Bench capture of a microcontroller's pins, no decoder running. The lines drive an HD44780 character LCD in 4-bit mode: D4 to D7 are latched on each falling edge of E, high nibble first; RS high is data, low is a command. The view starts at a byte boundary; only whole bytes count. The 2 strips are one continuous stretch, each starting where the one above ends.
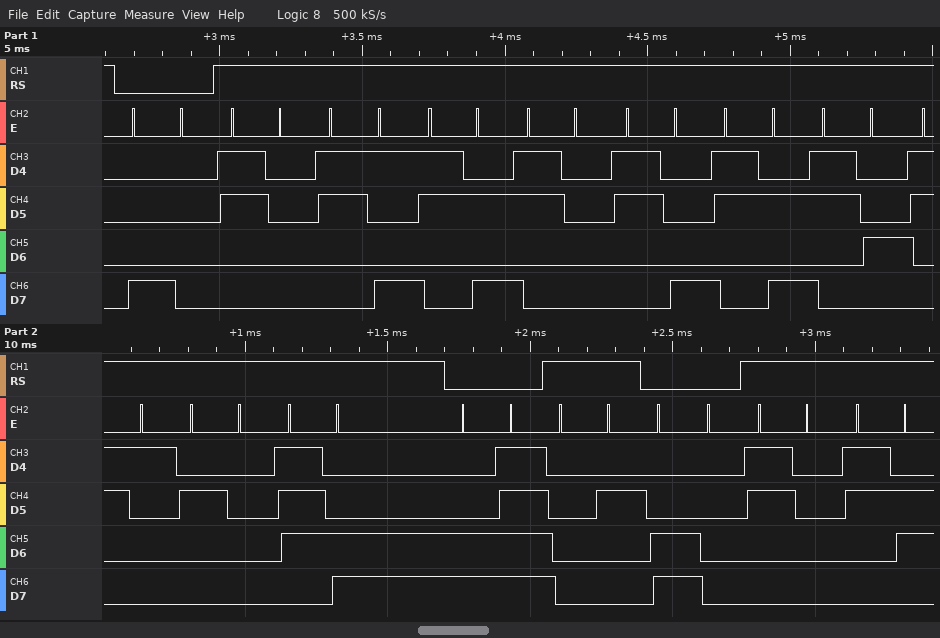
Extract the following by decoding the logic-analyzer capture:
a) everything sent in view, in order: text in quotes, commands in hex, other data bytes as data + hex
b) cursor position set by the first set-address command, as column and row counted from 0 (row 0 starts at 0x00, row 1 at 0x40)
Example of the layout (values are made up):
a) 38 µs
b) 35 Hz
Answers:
a) 0x80 "09:08:41 |" 0xCF data 02 0xC0 "06"
b) column 0, row 0
